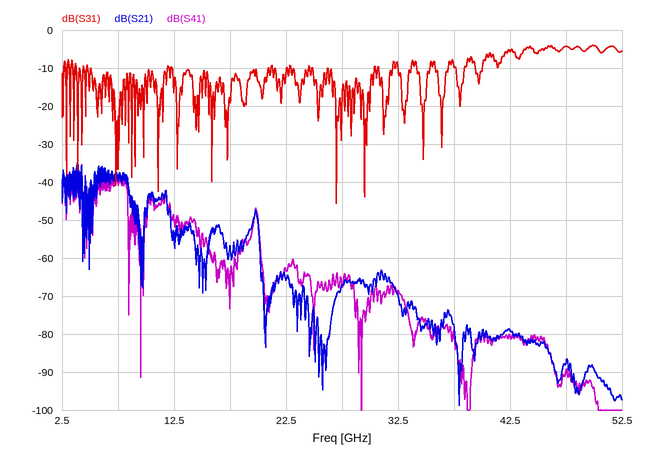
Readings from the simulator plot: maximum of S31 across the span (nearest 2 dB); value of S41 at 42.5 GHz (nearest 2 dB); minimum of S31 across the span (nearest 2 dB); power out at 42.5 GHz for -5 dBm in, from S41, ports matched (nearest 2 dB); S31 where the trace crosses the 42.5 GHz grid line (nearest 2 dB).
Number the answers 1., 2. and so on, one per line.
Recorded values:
1. -4 dB
2. -80 dB
3. -46 dB
4. -86 dBm
5. -6 dB
